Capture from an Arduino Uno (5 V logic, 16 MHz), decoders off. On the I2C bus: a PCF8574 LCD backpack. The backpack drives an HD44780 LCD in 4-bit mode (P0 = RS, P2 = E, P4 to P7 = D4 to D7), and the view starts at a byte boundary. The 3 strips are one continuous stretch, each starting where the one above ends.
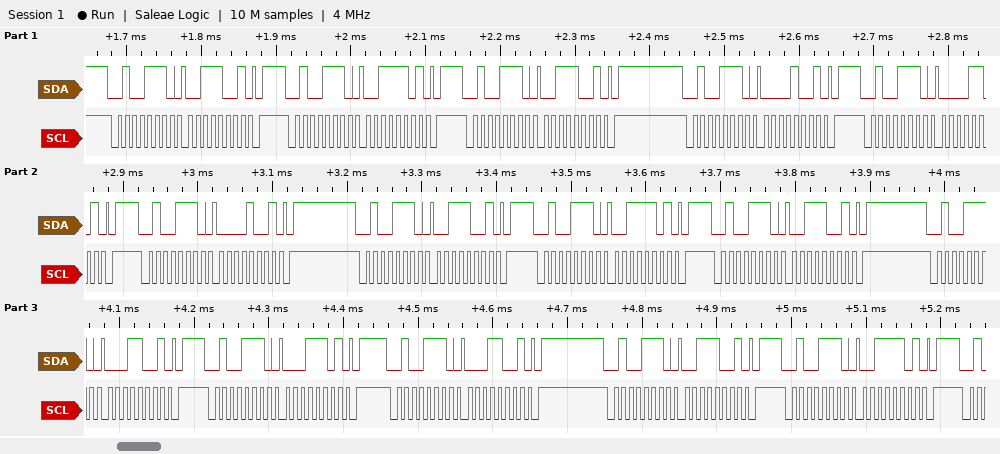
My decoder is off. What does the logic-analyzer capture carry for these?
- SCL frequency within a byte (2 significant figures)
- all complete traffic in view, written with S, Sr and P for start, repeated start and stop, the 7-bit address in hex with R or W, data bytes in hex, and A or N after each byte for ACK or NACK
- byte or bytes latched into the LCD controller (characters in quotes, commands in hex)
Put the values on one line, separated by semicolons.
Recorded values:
100 kHz; S 27W A 39 A P S 27W A 3D A P S 27W A 39 A P S 27W A 09 A P S 27W A 0D A P S 27W A 09 A P S 27W A 39 A P S 27W A 3D A P S 27W A 39 A P S 27W A 19 A P S 27W A 1D A P S 27W A 19 A P S 27W A 39 A P S 27W A 3D A P; '0' '1'
